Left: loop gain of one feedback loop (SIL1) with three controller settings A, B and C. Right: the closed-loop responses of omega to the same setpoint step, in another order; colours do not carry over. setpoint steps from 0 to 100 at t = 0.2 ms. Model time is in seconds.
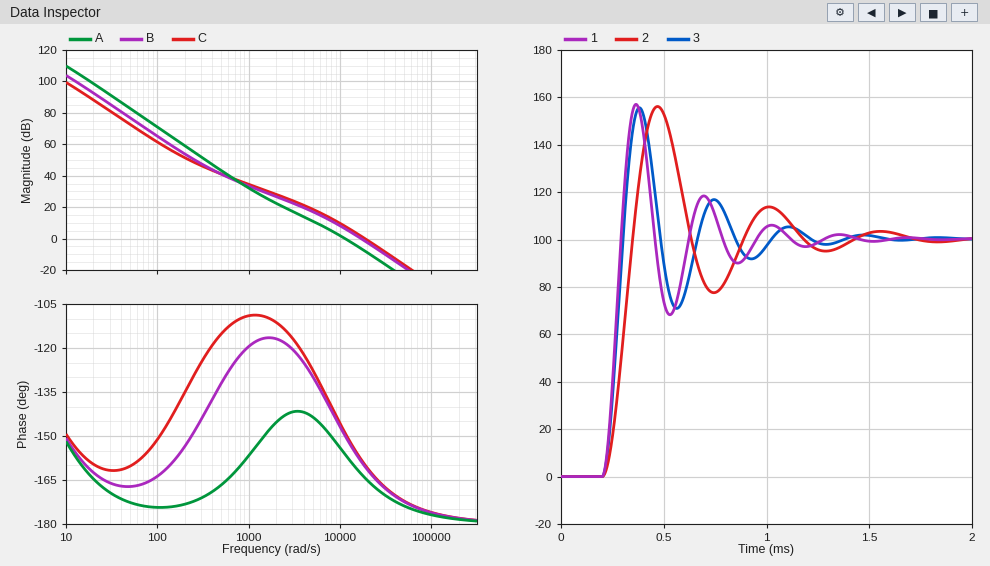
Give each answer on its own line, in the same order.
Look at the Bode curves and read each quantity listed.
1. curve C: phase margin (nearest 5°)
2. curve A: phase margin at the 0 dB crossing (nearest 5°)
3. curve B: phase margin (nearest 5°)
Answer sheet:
20°
25°
20°
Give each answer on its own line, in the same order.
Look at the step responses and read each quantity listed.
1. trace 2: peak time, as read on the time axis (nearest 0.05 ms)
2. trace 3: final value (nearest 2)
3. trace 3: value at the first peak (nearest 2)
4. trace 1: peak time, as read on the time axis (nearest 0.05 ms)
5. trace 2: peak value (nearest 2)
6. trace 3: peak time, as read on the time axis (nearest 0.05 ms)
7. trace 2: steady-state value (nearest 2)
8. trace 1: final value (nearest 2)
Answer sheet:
0.45 ms
100
156
0.35 ms
156
0.40 ms
100
100
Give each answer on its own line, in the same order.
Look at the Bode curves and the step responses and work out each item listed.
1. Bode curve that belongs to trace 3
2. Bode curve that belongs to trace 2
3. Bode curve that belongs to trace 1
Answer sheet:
B
A
C
